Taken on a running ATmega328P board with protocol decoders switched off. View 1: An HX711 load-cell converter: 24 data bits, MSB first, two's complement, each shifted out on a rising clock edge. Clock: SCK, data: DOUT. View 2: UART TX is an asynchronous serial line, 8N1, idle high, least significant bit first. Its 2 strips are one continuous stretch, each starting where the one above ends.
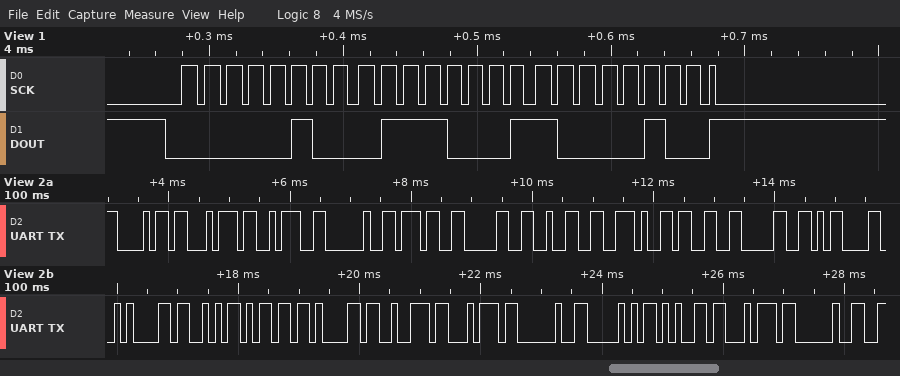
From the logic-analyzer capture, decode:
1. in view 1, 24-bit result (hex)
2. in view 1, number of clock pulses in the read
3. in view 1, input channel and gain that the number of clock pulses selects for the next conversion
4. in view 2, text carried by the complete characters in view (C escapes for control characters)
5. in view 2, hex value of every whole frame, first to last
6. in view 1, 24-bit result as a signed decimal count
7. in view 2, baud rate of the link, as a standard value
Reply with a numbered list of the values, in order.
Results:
1. 0x047184
2. 25
3. channel A, gain 128
4. "ht: 702.30\r\nSmart Pet "
5. 68 74 3A 20 37 30 32 2E 33 30 0D 0A 53 6D 61 72 74 20 50 65 74 20
6. 291204
7. 9600 baud
